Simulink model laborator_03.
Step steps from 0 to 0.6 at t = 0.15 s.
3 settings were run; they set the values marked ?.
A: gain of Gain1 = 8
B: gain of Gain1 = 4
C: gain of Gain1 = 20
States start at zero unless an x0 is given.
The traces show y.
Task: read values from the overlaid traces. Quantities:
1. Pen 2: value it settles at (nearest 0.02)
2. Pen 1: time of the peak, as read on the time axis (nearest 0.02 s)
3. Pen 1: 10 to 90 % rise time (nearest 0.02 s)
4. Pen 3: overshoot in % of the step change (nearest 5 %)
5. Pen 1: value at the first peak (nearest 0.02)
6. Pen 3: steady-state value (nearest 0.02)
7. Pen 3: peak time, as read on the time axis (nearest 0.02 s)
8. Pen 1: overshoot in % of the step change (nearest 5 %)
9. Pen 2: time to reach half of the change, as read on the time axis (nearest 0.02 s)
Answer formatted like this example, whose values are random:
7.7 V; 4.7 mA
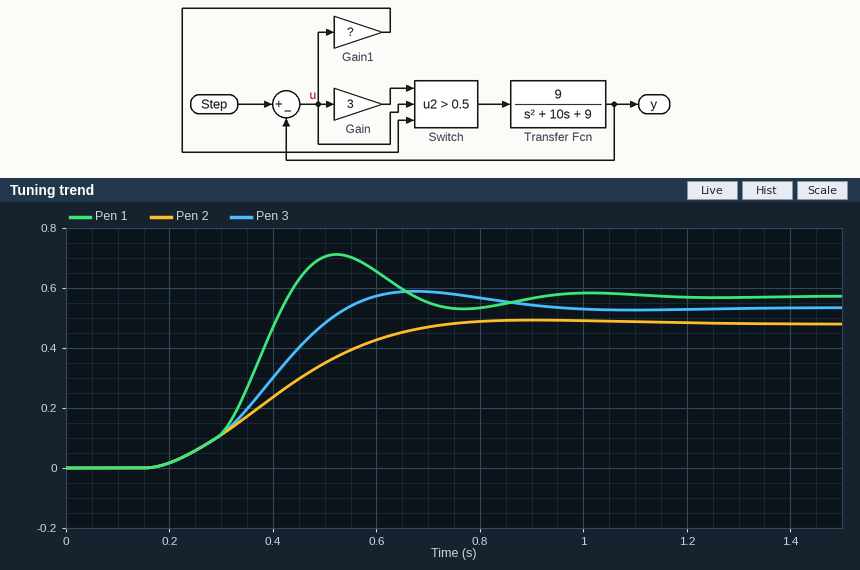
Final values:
0.48; 0.52 s; 0.16 s; 10 %; 0.72; 0.54; 0.68 s; 25 %; 0.40 s
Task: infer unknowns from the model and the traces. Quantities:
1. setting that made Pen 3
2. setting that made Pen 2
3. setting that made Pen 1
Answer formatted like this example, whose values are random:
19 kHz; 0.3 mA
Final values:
A; B; C
